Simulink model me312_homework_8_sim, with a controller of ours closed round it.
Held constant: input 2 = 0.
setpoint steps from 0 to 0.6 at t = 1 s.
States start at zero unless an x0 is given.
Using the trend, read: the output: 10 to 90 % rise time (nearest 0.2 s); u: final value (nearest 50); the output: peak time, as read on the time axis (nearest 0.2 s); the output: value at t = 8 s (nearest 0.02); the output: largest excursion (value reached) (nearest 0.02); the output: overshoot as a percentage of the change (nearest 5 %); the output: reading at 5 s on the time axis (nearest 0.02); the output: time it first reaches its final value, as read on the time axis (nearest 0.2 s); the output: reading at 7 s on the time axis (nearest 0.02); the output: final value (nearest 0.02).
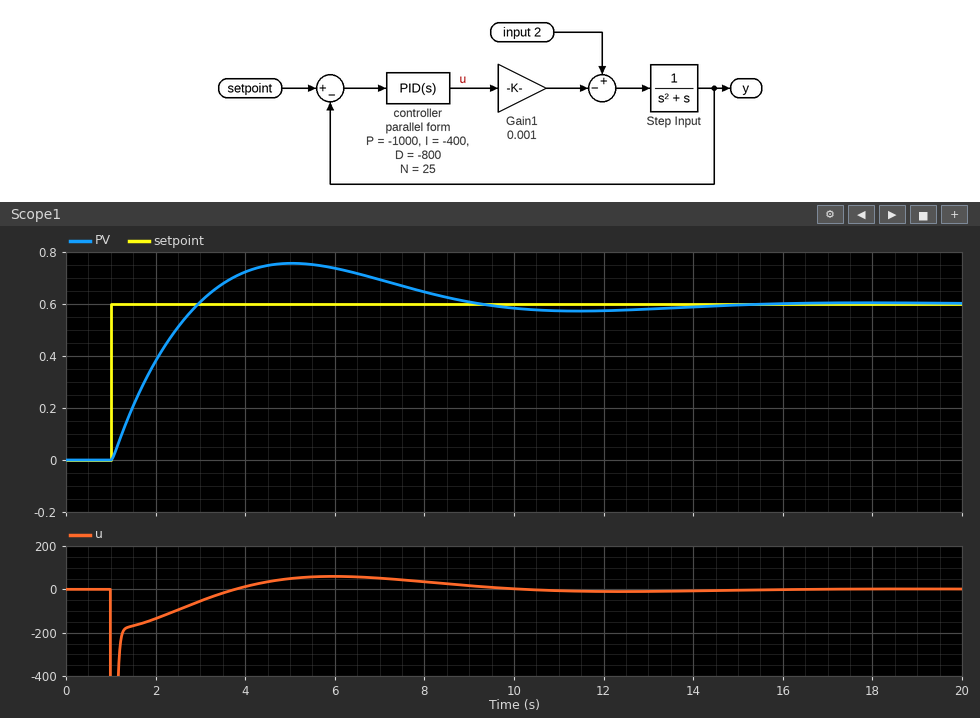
1.4 s
0
5.0 s
0.64
0.76
25 %
0.76
3.0 s
0.70
0.60
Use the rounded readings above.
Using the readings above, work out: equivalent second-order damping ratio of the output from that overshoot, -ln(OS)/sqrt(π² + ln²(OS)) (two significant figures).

0.40
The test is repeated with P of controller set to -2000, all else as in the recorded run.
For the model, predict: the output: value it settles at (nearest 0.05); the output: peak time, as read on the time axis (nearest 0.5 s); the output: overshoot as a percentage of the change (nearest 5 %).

0.60
3.5 s
20 %
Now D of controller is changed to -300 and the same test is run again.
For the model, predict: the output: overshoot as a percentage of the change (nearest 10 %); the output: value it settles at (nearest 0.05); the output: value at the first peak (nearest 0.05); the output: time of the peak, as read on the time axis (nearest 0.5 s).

40 %
0.60
0.85
4.5 s
